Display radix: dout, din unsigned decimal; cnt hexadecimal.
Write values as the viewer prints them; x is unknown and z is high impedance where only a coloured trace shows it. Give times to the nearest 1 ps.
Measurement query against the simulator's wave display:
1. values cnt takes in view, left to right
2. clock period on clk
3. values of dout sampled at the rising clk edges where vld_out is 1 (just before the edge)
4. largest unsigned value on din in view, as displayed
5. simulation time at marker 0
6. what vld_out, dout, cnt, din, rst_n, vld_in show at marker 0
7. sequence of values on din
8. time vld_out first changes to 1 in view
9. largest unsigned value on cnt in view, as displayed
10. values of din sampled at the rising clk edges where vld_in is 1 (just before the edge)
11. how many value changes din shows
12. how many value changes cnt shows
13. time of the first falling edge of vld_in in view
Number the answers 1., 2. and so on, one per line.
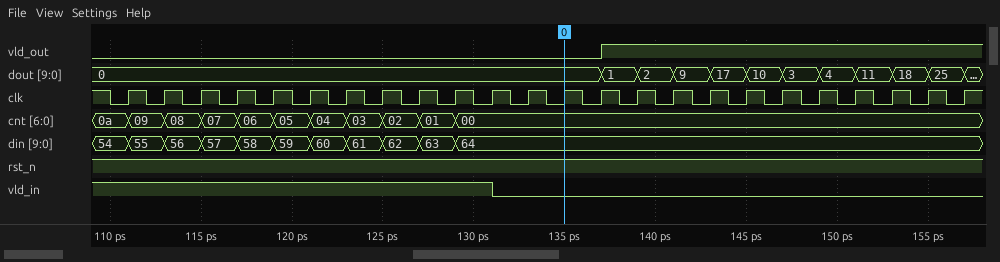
1. 0a, 09, 08, 07, 06, 05, 04, 03, 02, 01, 00
2. 2 ps
3. 1, 2, 9, 17, 10, 3, 4, 11, 18, 25
4. 64
5. 135 ps
6. vld_out=0, dout=0, cnt=00, din=64, rst_n=1, vld_in=0
7. 54, 55, 56, 57, 58, 59, 60, 61, 62, 63, 64
8. 137 ps
9. 0a
10. 54, 55, 56, 57, 58, 59, 60, 61, 62, 63, 64
11. 10
12. 10
13. 131 ps
